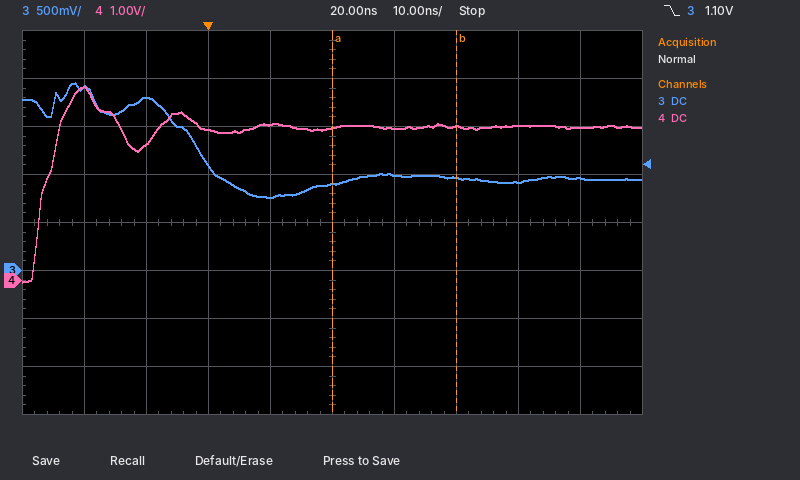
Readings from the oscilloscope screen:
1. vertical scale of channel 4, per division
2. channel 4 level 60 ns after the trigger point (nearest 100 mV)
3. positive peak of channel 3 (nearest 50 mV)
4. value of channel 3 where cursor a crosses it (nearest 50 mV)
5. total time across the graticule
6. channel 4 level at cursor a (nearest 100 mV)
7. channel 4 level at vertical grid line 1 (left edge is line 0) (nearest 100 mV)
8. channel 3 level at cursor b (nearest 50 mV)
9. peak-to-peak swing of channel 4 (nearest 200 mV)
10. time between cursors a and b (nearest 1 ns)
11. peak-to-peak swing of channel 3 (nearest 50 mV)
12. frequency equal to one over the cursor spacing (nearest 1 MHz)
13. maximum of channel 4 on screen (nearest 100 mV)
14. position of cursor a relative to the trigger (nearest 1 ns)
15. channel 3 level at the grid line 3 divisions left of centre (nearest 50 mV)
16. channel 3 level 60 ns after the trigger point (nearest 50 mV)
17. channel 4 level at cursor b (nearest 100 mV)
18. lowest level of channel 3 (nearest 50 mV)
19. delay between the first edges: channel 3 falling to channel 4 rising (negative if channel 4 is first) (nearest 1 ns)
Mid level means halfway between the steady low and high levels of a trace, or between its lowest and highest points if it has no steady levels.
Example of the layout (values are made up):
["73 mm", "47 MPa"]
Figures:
["1 V", "3.2 V", "1.95 V", "900 mV", "100 ns", "3.2 V", "4.0 V", "950 mV", "4.0 V", "20 ns", "1.20 V", "50 MHz", "4.0 V", "+20 ns", "1.80 V", "950 mV", "3.2 V", "750 mV", "-24 ns"]
